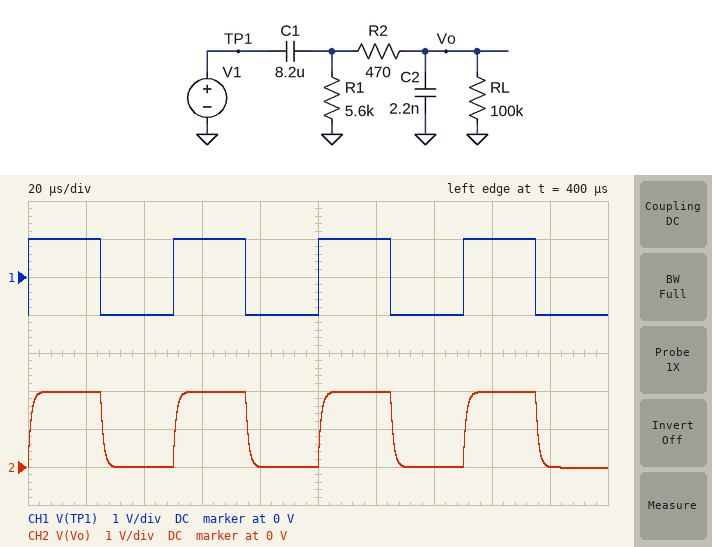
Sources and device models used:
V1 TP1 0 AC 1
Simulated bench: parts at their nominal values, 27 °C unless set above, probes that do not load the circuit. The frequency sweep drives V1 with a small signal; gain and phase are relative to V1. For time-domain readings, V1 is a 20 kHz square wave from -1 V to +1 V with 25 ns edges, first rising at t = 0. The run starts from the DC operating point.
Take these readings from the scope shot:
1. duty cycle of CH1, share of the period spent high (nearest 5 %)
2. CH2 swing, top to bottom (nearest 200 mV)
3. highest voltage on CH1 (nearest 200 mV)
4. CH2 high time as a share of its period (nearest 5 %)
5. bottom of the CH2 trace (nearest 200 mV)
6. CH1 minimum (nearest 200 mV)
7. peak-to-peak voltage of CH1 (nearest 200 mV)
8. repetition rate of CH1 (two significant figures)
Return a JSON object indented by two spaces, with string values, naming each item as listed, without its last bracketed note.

{
  "duty cycle of CH1, share of the period spent high": "50 %",
  "CH2 swing, top to bottom": "2.0 V",
  "highest voltage on CH1": "1.0 V",
  "CH2 high time as a share of its period": "50 %",
  "bottom of the CH2 trace": "0 V",
  "CH1 minimum": "-1.0 V",
  "peak-to-peak voltage of CH1": "2.0 V",
  "repetition rate of CH1": "20 kHz"
}
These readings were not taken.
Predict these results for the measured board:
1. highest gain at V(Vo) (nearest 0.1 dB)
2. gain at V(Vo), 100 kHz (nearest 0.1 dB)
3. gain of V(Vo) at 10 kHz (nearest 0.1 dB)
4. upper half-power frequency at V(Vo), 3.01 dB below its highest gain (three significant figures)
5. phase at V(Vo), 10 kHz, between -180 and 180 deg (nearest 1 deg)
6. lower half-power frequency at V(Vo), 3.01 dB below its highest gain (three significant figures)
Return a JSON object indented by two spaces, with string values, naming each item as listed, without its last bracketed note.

{
  "highest gain at V(Vo)": "0 dB",
  "gain at V(Vo), 100 kHz": "-1.6 dB",
  "gain of V(Vo) at 10 kHz": "-0.1 dB",
  "upper half-power frequency at V(Vo), 3.01 dB below its highest gain": "155 kHz",
  "phase at V(Vo), 10 kHz, between -180 and 180 deg": "-4 deg",
  "lower half-power frequency at V(Vo), 3.01 dB below its highest gain": "3.66 Hz"
}
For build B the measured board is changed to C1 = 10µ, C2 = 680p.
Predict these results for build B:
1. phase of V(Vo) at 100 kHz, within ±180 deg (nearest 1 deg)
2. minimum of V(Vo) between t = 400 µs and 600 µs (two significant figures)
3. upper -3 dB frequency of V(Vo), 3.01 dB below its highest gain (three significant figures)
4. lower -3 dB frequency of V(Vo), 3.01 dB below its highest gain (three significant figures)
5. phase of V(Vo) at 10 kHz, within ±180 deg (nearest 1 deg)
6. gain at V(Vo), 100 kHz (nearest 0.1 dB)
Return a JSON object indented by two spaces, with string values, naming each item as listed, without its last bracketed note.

{
  "phase of V(Vo) at 100 kHz, within ±180 deg": "-11 deg",
  "minimum of V(Vo) between t = 400 µs and 600 µs": "-11 mV",
  "upper -3 dB frequency of V(Vo), 3.01 dB below its highest gain": "500 kHz",
  "lower -3 dB frequency of V(Vo), 3.01 dB below its highest gain": "3.00 Hz",
  "phase of V(Vo) at 10 kHz, within ±180 deg": "-1 deg",
  "gain at V(Vo), 100 kHz": "-0.2 dB"
}
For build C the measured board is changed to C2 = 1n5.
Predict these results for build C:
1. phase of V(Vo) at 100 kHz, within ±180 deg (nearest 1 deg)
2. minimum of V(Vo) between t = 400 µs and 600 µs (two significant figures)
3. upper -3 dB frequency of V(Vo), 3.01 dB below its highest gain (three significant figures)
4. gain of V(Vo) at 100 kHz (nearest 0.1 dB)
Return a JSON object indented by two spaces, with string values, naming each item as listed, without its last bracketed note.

{
  "phase of V(Vo) at 100 kHz, within ±180 deg": "-24 deg",
  "minimum of V(Vo) between t = 400 µs and 600 µs": "-14 mV",
  "upper -3 dB frequency of V(Vo), 3.01 dB below its highest gain": "227 kHz",
  "gain of V(Vo) at 100 kHz": "-0.8 dB"
}
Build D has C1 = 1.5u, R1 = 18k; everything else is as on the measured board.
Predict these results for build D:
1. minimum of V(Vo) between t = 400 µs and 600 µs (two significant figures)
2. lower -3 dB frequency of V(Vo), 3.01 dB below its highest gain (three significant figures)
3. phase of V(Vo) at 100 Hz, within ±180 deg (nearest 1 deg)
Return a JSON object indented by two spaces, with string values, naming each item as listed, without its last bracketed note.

{
  "minimum of V(Vo) between t = 400 µs and 600 µs": "-26 mV",
  "lower -3 dB frequency of V(Vo), 3.01 dB below its highest gain": "6.94 Hz",
  "phase of V(Vo) at 100 Hz, within ±180 deg": "4 deg"
}
